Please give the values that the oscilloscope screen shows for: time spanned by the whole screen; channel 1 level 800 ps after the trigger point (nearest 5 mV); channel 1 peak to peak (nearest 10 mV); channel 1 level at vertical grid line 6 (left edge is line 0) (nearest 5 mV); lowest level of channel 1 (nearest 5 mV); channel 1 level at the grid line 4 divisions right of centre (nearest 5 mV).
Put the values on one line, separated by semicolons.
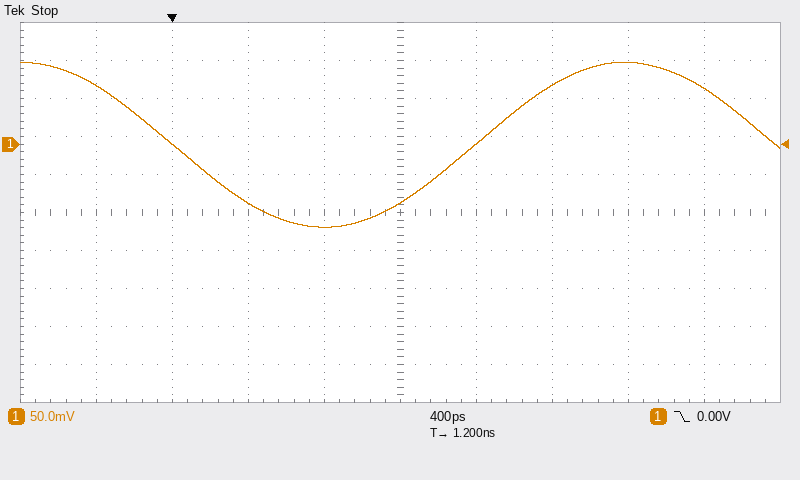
4 ns; -110 mV; 220 mV; 0 mV; -110 mV; 75 mV
